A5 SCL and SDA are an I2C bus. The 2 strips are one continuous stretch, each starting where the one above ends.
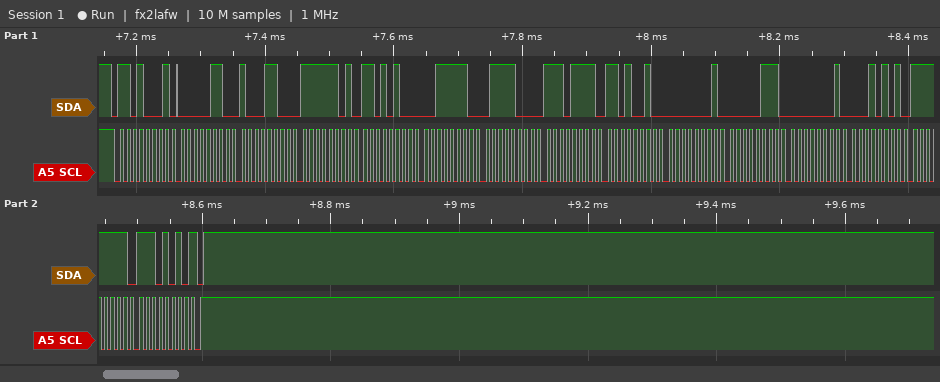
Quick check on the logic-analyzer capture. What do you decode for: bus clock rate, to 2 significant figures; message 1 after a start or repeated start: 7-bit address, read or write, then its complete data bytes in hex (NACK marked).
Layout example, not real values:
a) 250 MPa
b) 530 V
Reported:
a) 100 kHz
b) 0x68 read: 06 8C FD D4 3E 78 EF D2 01 07 01 15 FF EA NACK
